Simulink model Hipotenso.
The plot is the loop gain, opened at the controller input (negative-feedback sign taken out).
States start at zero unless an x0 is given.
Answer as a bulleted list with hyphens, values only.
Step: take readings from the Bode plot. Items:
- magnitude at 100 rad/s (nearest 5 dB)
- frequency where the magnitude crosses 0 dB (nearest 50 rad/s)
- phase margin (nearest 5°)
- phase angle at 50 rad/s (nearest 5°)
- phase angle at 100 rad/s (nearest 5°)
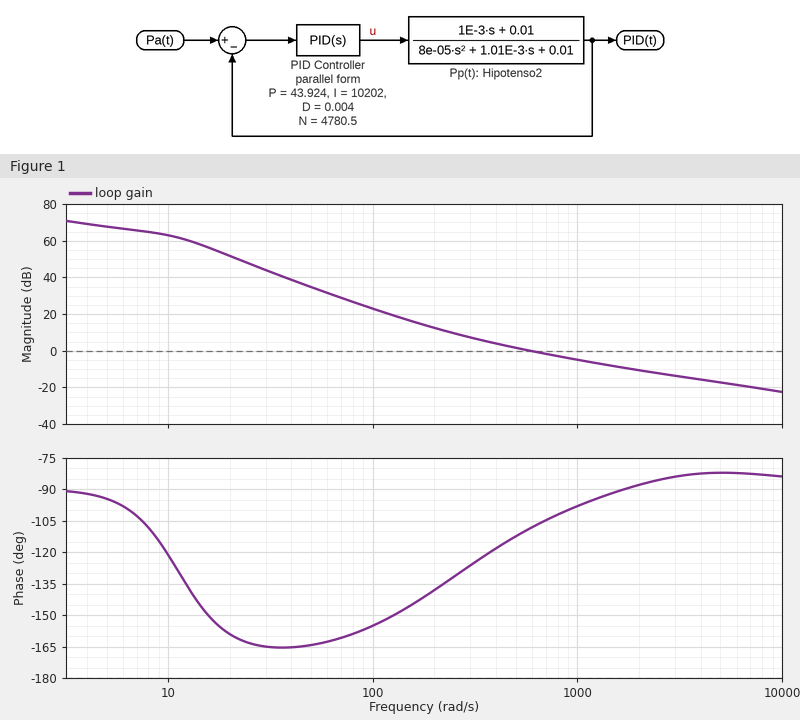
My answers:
- 25 dB
- 600 rad/s
- 70°
- -165°
- -155°
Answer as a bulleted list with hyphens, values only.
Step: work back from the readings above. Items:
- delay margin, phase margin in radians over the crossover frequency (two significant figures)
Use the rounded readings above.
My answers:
- 0.0020 s
